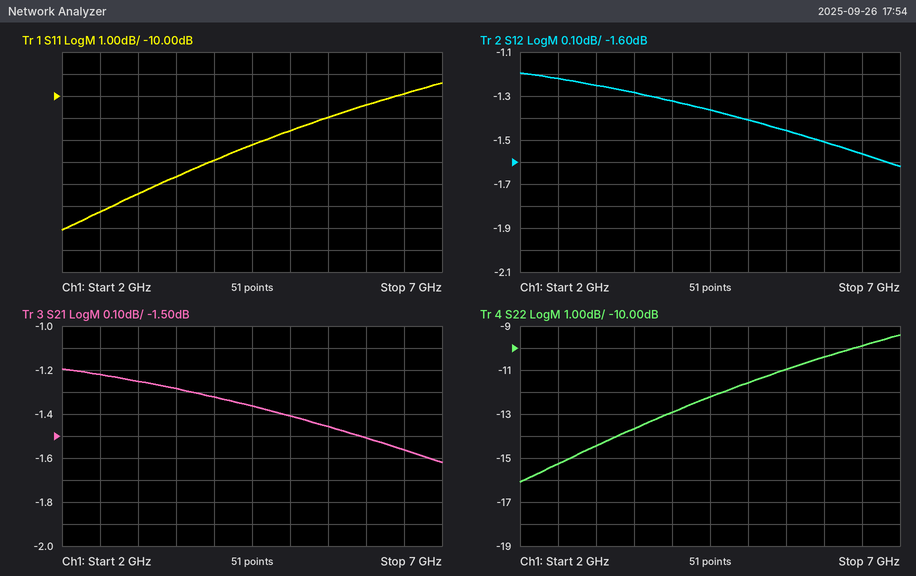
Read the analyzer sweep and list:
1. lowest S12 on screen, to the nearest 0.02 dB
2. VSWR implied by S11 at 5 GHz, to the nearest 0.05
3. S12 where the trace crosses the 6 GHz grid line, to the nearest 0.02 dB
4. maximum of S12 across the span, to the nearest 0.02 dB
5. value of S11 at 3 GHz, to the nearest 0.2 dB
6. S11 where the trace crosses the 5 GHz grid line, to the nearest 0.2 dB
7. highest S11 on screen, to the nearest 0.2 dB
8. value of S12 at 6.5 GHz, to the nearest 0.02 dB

-1.62 dB
1.70
-1.50 dB
-1.20 dB
-14.4 dB
-11.6 dB
-9.4 dB
-1.56 dB
